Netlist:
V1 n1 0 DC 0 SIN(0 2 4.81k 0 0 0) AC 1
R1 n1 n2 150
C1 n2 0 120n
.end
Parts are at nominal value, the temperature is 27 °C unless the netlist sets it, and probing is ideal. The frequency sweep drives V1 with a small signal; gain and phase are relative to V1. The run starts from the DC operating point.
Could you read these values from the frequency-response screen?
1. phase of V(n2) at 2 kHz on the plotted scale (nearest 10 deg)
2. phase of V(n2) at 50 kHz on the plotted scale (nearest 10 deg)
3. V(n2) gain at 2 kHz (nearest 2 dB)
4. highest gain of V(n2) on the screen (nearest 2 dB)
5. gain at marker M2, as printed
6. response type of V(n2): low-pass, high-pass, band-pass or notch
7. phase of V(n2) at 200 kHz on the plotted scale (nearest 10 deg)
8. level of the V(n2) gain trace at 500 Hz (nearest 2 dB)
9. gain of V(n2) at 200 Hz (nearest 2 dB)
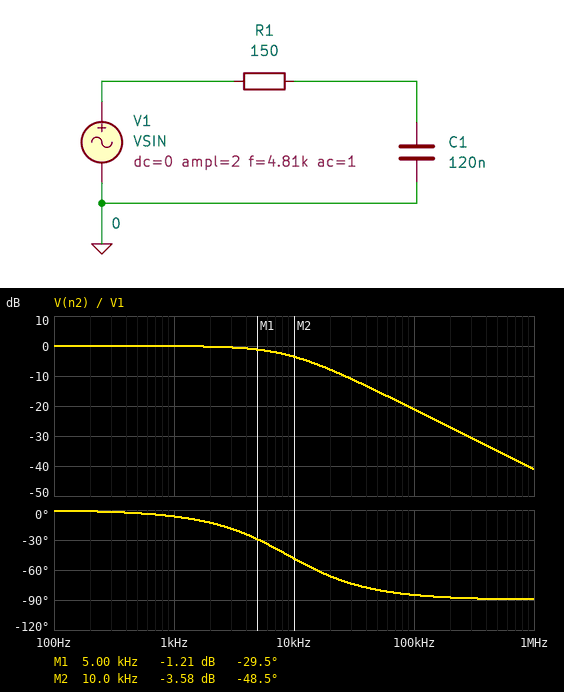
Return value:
-10 deg
-80 deg
0 dB
0 dB
-3.58 dB
low-pass
-90 deg
0 dB
0 dB
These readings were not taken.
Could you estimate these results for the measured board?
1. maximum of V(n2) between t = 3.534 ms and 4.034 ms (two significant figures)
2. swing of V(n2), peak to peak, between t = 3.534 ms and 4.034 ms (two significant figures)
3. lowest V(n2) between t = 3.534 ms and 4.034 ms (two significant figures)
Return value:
1.8 V
3.5 V
-1.8 V
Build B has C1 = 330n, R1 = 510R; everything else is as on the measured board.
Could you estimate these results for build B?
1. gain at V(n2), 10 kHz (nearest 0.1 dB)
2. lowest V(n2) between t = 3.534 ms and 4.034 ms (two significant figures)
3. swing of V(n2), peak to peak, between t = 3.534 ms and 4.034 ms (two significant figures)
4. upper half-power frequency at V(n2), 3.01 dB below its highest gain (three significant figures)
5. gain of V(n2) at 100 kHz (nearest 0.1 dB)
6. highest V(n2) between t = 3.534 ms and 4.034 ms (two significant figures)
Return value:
-20.5 dB
-390 mV
770 mV
946 Hz
-40.5 dB
390 mV
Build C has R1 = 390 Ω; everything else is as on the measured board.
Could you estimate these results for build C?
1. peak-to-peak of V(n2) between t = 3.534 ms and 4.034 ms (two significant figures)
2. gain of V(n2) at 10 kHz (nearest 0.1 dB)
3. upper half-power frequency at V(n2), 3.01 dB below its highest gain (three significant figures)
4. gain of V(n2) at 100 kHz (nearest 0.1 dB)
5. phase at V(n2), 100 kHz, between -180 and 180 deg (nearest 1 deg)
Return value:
2.3 V
-9.8 dB
3.40 kHz
-29.4 dB
-88 deg
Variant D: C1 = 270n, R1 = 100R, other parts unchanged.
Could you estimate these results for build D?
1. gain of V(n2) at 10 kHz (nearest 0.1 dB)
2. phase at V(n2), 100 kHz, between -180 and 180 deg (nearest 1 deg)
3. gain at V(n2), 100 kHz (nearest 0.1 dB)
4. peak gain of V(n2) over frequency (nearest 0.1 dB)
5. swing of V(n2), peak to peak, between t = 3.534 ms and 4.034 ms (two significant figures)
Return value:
-5.9 dB
-87 deg
-24.6 dB
0 dB
3.1 V
